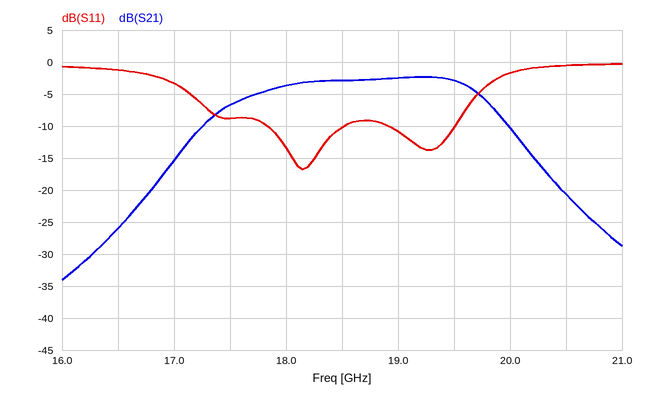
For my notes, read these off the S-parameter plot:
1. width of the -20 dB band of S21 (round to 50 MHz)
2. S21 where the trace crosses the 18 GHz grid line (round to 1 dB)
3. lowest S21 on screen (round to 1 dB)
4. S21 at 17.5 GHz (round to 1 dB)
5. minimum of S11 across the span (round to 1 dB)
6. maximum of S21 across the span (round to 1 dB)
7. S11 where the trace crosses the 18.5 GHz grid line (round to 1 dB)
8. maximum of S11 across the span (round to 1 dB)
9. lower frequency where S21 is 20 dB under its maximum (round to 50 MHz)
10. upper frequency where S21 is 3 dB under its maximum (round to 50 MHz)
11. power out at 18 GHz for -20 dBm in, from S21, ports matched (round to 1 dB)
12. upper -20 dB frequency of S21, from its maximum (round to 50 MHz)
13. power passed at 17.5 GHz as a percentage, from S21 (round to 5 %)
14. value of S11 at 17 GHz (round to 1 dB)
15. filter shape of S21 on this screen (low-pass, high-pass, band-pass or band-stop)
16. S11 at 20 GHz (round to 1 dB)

3.90 GHz
-4 dB
-34 dB
-7 dB
-17 dB
-2 dB
-10 dB
0 dB
16.70 GHz
19.75 GHz
-24 dBm
20.60 GHz
20 %
-3 dB
band-pass
-2 dB
